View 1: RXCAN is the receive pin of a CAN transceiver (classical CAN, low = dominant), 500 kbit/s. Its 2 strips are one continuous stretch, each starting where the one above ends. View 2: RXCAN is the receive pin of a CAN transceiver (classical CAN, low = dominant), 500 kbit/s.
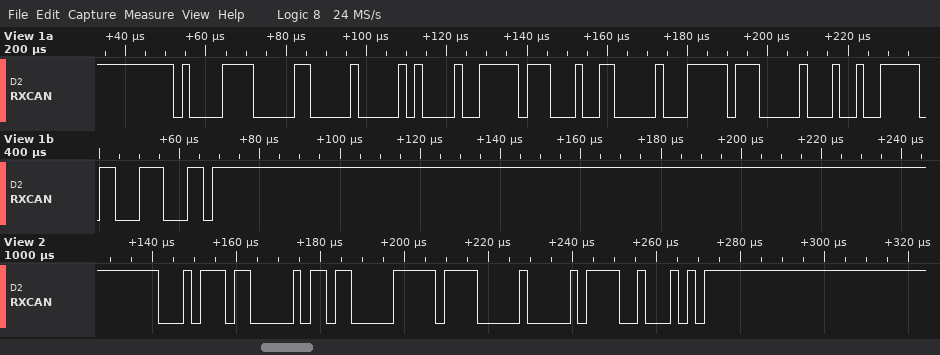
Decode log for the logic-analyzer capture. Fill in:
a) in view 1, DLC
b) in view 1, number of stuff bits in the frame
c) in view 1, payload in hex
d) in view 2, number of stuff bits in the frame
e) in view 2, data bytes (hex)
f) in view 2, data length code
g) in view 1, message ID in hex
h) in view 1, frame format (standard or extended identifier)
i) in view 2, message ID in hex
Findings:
8
8
00 84 FF 13 00 FF 00 93
5
60 FF 00
3
0x43C
standard
0x176
